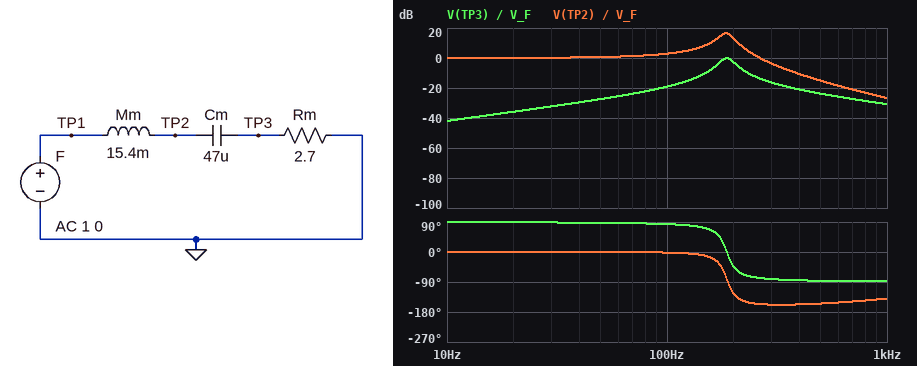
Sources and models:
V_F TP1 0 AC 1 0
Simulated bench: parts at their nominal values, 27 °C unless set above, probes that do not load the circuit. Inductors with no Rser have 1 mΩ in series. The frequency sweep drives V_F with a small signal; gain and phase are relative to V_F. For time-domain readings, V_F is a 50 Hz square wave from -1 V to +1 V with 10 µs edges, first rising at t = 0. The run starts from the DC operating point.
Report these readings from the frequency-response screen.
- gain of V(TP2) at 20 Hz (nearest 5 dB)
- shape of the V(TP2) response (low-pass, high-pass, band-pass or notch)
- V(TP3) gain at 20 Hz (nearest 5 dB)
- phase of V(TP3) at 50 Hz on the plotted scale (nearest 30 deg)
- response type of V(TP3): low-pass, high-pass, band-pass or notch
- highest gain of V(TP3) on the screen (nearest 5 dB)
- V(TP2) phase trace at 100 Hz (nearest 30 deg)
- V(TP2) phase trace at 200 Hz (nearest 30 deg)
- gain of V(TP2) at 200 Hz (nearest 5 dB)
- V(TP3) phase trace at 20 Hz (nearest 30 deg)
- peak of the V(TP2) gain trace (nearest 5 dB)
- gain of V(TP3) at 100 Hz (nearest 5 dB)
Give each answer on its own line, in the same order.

0 dB
low-pass
-35 dB
90 deg
band-pass
0 dB
0 deg
-120 deg
15 dB
90 deg
15 dB
-20 dB
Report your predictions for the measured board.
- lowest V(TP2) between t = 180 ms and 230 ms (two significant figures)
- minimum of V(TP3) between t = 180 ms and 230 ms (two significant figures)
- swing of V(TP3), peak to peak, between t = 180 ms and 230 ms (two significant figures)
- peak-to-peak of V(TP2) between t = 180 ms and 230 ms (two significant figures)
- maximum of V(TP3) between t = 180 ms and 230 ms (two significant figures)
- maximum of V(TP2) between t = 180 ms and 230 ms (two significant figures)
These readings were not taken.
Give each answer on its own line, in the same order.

-2.2 V
-210 mV
410 mV
4.5 V
210 mV
2.2 V
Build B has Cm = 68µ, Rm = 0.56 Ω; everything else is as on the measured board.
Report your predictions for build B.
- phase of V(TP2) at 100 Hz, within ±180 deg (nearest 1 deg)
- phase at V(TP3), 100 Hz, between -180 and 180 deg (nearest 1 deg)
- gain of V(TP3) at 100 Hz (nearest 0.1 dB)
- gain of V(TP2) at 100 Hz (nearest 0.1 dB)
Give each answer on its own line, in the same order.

-1 deg
88 deg
-27.8 dB
4.6 dB
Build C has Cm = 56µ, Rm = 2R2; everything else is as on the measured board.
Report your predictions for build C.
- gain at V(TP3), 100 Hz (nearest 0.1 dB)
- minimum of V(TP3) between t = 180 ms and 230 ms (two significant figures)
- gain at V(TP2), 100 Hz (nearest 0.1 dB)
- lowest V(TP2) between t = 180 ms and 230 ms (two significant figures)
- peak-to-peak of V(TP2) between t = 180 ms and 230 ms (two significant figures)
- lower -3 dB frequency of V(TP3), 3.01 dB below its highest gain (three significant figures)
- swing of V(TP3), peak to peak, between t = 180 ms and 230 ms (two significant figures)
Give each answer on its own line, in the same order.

-18.7 dB
-250 mV
3.6 dB
-2.7 V
5.4 V
160 Hz
500 mV
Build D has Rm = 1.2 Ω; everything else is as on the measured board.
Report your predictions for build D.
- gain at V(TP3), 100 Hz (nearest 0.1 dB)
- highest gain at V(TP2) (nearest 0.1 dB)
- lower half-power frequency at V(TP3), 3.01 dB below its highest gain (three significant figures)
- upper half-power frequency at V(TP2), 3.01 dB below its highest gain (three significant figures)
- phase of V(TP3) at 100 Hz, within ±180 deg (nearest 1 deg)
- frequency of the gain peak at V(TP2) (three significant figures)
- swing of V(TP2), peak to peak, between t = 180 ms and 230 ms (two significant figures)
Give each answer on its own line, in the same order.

-26.1 dB
23.6 dB
181 Hz
193 Hz
87 deg
187 Hz
4.4 V
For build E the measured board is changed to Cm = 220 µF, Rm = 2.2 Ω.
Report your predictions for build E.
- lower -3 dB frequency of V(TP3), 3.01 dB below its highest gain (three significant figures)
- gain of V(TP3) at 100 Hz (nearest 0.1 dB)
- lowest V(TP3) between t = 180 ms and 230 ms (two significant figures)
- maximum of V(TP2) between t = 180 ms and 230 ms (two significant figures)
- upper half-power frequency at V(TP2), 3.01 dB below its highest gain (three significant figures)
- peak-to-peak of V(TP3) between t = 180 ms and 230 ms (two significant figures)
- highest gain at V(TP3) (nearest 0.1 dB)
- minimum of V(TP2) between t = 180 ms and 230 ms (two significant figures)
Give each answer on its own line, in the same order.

75.8 Hz
-3.5 dB
-330 mV
2.0 V
95.9 Hz
660 mV
0 dB
-2.0 V
